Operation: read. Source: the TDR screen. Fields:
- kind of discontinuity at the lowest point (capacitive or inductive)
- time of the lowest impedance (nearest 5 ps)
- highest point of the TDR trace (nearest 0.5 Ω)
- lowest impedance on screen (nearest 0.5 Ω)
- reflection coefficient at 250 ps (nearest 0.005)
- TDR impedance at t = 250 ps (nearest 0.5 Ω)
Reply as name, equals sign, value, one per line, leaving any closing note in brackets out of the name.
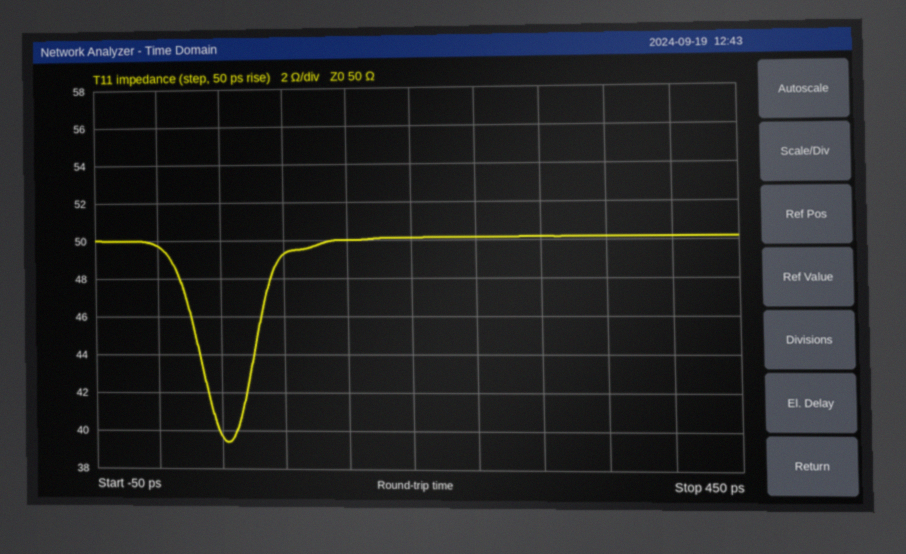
kind of discontinuity at the lowest point = capacitive
time of the lowest impedance = 55 ps
highest point of the TDR trace = 50.0 Ω
lowest impedance on screen = 39.5 Ω
reflection coefficient at 250 ps = 0.000
TDR impedance at t = 250 ps = 50.0 Ω
